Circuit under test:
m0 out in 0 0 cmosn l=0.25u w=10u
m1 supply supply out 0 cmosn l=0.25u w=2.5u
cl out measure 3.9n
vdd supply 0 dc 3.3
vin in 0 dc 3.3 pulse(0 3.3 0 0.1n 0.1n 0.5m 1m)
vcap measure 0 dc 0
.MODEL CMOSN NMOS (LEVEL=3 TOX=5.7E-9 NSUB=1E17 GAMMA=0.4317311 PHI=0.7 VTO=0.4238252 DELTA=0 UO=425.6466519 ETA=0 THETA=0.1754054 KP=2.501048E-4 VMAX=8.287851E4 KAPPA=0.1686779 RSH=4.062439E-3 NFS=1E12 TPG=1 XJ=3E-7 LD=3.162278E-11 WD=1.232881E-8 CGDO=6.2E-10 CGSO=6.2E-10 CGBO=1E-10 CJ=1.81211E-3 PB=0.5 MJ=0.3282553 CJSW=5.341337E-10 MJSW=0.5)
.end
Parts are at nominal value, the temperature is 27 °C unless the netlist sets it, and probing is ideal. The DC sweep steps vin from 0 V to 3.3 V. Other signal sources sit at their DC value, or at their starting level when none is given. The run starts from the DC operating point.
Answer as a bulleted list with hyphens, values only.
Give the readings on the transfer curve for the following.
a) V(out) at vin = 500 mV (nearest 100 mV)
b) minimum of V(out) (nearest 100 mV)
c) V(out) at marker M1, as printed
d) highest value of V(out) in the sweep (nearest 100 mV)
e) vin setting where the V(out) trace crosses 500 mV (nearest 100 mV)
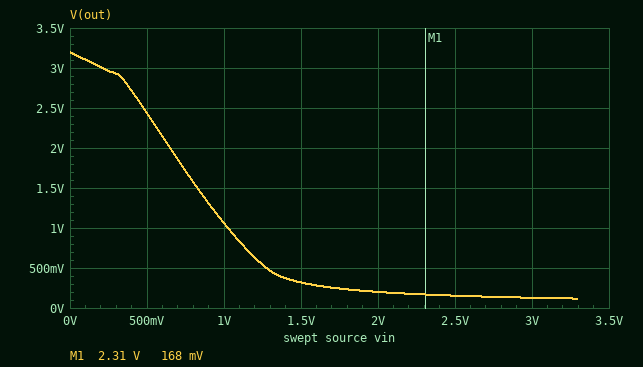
- 2.4 V
- 100 mV
- 168 mV
- 3.2 V
- 1.3 V
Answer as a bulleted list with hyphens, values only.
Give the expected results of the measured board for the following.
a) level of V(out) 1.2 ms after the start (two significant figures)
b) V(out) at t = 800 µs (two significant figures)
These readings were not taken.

- 120 mV
- 3.0 V
